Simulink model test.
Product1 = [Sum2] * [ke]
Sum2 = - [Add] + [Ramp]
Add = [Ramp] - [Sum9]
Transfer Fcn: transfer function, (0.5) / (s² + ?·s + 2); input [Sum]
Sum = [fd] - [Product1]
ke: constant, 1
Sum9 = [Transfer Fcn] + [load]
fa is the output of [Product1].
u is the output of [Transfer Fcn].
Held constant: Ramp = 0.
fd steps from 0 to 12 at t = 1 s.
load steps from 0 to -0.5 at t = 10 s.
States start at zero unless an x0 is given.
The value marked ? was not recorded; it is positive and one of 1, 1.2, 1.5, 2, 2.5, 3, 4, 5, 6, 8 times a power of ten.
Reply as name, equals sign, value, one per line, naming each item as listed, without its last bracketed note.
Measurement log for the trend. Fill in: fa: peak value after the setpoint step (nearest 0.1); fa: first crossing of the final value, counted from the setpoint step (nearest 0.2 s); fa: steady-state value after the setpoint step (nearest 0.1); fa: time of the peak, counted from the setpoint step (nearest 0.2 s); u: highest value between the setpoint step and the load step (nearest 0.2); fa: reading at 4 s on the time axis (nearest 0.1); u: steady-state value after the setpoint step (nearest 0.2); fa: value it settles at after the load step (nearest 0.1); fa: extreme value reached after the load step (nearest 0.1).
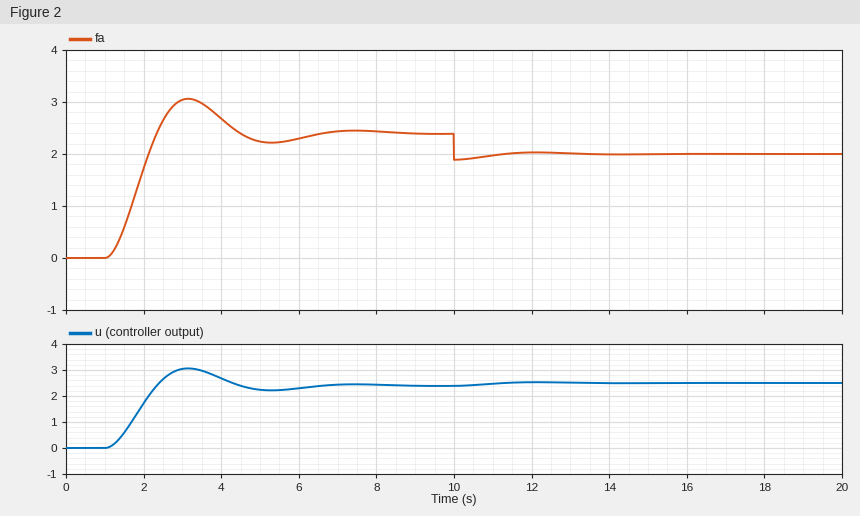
fa: peak value after the setpoint step = 3.1
fa: first crossing of the final value, counted from the setpoint step = 1.4 s
fa: steady-state value after the setpoint step = 2.4
fa: time of the peak, counted from the setpoint step = 2.2 s
u: highest value between the setpoint step and the load step = 3.0
fa: reading at 4 s on the time axis = 2.7
u: steady-state value after the setpoint step = 2.4
fa: value it settles at after the load step = 2.0
fa: extreme value reached after the load step = 1.9
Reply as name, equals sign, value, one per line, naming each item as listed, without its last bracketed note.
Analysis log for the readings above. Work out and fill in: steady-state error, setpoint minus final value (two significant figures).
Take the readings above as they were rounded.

steady-state error, setpoint minus final value = 9.6
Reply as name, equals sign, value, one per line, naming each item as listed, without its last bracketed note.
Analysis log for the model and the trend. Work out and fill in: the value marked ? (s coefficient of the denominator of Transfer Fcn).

the value marked ? = 1.2
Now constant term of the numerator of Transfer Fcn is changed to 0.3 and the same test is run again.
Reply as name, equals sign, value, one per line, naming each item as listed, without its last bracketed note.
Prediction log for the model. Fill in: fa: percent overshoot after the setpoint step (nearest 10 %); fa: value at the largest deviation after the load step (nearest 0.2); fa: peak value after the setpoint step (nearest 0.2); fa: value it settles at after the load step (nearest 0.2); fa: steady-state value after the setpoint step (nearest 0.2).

fa: percent overshoot after the setpoint step = 30 %
fa: value at the largest deviation after the load step = 1.0
fa: peak value after the setpoint step = 2.0
fa: value it settles at after the load step = 1.2
fa: steady-state value after the setpoint step = 1.6
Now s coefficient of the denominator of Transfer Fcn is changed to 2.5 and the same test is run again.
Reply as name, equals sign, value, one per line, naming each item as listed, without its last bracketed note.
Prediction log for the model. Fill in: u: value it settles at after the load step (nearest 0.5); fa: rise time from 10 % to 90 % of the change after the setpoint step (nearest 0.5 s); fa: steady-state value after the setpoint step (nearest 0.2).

u: value it settles at after the load step = 2.5
fa: rise time from 10 % to 90 % of the change after the setpoint step = 1.5 s
fa: steady-state value after the setpoint step = 2.4
